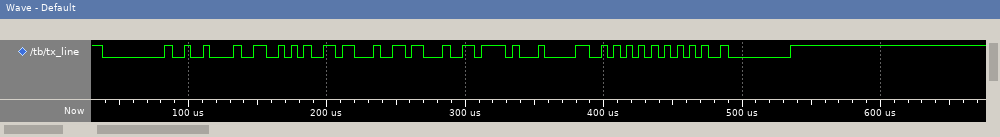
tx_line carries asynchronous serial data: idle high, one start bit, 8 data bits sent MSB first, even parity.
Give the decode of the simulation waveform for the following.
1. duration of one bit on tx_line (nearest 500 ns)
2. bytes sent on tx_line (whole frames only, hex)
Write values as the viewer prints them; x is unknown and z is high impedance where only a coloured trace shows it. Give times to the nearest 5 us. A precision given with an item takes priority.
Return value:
4500 ns
00, 48, 65, 6C, 6C, 6F, 20, 55, AA, 00
